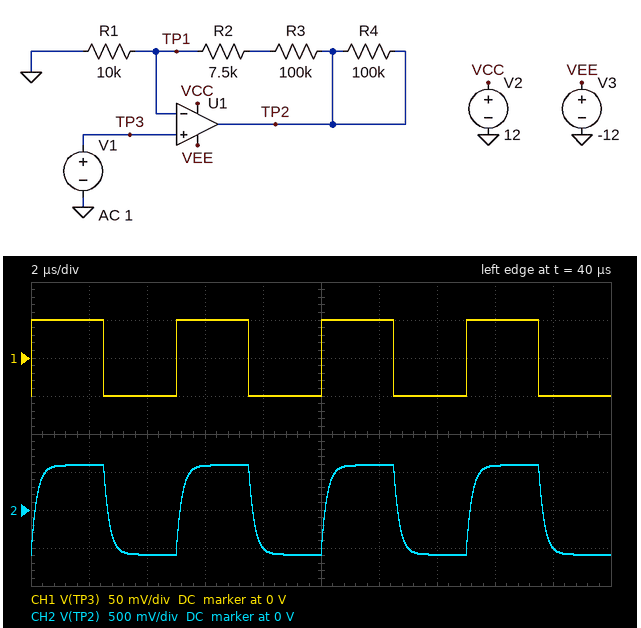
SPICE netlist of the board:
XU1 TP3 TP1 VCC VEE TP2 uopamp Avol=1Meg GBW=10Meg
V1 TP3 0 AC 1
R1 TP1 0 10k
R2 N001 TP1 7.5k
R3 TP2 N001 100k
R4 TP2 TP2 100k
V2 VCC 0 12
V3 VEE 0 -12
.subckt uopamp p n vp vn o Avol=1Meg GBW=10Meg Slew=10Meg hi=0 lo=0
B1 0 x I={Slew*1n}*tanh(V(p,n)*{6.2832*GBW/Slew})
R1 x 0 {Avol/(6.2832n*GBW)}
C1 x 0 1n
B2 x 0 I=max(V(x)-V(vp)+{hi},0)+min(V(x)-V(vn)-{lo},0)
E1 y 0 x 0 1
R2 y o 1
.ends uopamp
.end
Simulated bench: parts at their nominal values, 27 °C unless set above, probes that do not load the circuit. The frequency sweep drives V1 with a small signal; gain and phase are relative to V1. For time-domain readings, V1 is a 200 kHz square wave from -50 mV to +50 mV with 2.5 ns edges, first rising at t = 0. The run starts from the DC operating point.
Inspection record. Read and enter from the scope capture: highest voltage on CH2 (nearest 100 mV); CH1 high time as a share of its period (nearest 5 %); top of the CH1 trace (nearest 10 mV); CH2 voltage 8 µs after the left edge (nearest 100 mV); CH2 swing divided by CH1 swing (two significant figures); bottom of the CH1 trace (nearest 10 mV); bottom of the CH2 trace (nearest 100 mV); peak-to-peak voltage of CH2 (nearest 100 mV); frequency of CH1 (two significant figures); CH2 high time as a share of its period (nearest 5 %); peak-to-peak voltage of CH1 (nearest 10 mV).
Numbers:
600 mV
50 %
50 mV
-500 mV
12
-50 mV
-600 mV
1.2 V
200 kHz
50 %
100 mV
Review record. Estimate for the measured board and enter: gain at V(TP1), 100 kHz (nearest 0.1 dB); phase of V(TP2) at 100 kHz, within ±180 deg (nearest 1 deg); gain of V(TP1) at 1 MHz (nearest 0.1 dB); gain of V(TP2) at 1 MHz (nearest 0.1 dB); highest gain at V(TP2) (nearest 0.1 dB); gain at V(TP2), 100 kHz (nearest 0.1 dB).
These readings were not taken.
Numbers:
-0.1 dB
-7 deg
-3.8 dB
17.6 dB
21.4 dB
21.3 dB
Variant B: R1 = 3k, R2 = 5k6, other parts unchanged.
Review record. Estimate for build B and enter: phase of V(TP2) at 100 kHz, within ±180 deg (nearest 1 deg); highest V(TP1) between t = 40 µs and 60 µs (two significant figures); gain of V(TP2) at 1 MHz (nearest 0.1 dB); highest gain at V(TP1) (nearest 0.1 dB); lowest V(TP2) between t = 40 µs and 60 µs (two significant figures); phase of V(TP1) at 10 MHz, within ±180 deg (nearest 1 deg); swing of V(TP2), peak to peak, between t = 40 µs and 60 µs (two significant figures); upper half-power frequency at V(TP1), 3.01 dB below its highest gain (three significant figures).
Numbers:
-20 deg
49 mV
19.7 dB
0 dB
-1.8 V
-88 deg
3.5 V
276 kHz
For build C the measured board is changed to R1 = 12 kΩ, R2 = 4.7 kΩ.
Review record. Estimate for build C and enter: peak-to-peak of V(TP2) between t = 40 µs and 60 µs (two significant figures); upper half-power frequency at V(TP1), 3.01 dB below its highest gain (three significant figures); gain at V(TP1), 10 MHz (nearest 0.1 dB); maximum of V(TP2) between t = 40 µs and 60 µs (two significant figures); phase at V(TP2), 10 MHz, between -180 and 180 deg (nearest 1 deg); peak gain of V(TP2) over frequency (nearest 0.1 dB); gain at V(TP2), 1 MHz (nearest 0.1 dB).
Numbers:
970 mV
1.03 MHz
-19.8 dB
490 mV
-84 deg
19.8 dB
16.9 dB
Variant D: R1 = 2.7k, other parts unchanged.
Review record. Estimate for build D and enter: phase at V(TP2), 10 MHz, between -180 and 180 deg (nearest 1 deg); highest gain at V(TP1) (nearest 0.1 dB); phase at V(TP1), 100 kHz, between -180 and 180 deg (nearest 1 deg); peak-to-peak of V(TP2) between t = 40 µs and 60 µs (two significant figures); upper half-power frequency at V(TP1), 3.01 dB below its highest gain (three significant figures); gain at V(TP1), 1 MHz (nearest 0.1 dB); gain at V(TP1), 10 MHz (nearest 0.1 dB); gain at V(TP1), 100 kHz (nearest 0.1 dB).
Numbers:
-89 deg
0 dB
-22 deg
3.9 V
245 kHz
-12.5 dB
-32.2 dB
-0.7 dB
